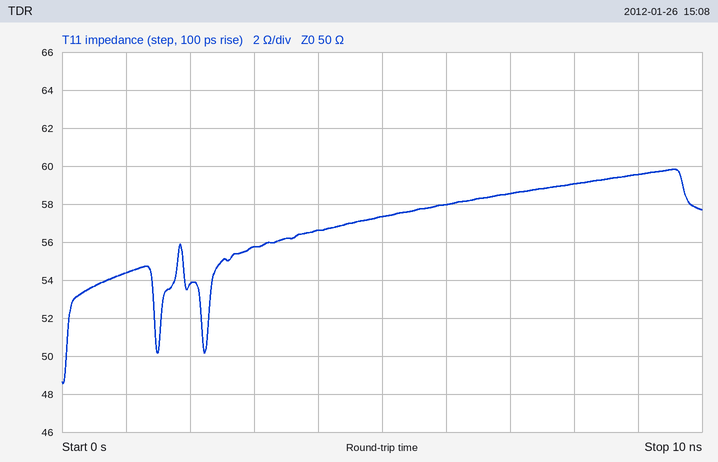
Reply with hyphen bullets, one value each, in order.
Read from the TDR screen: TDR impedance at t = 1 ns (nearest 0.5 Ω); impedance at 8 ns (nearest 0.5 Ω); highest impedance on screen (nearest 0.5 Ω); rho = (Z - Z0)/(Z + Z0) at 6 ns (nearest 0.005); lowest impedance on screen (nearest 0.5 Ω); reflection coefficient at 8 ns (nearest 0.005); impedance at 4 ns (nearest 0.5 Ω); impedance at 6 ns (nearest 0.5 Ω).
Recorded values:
- 54.5 Ω
- 59.0 Ω
- 60.0 Ω
- +0.075
- 48.5 Ω
- +0.085
- 56.5 Ω
- 58.0 Ω
